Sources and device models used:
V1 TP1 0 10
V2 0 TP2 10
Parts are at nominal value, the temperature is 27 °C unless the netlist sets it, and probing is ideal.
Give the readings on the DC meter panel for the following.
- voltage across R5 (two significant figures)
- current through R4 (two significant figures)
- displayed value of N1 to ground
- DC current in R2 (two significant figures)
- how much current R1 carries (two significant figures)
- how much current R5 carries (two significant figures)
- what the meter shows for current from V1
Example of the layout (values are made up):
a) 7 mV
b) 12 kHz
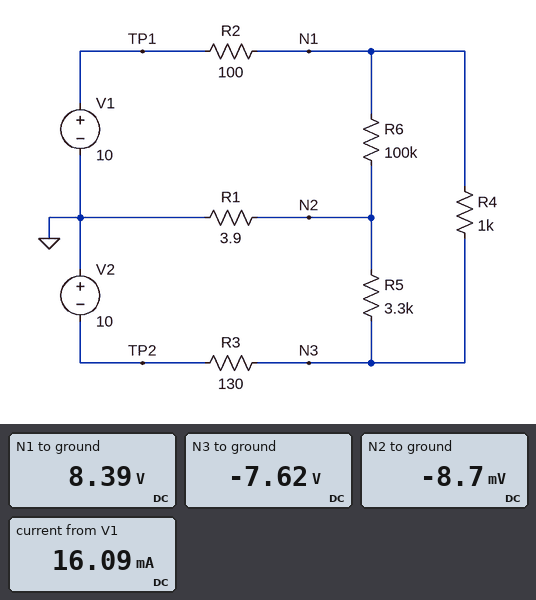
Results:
a) 7.6 V
b) 16 mA
c) 8.39 V
d) 16 mA
e) 2.2 mA
f) 2.3 mA
g) 16.09 mA
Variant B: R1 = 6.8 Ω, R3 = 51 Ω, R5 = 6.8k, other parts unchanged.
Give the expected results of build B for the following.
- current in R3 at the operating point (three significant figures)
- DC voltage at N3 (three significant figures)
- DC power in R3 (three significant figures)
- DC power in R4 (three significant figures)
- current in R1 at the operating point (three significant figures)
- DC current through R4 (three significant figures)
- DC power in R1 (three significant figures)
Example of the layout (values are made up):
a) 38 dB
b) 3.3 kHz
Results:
a) 18.6 mA
b) -9.05 V
c) 17.7 mW
d) 300 mW
e) 1.25 mA
f) 17.3 mA
g) 10.6 µW
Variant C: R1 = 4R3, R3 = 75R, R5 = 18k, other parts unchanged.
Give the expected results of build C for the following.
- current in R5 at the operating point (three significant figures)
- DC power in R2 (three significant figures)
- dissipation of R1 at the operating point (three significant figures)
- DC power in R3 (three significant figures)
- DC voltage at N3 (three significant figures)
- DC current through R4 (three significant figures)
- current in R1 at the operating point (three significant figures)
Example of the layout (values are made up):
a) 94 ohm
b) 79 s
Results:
a) 483 µA
b) 29.1 mW
c) 687 nW
d) 22.9 mW
e) -8.69 V
f) 17.0 mA
g) 400 µA
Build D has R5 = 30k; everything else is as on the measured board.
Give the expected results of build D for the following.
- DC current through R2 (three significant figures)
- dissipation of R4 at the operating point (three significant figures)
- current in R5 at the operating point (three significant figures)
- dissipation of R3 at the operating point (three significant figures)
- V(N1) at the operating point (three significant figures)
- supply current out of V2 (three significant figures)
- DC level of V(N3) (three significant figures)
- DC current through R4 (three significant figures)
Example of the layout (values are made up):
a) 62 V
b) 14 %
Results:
a) 16.3 mA
b) 263 mW
c) 262 µA
d) 35.3 mW
e) 8.37 V
f) 16.5 mA
g) -7.86 V
h) 16.2 mA
